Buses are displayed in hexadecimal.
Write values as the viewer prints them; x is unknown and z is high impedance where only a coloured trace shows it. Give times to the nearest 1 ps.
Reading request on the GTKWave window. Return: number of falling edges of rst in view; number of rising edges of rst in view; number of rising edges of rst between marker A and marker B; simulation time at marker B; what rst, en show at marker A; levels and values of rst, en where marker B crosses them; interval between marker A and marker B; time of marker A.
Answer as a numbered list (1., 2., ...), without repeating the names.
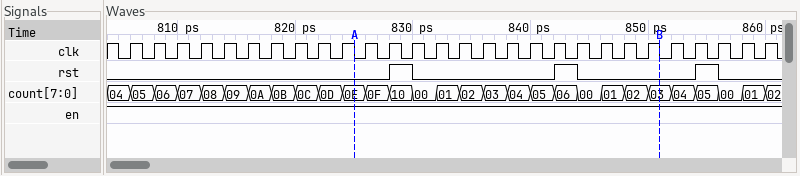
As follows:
1. 3
2. 3
3. 2
4. 851 ps
5. rst=0, en=1
6. rst=0, en=1
7. 26 ps
8. 825 ps
